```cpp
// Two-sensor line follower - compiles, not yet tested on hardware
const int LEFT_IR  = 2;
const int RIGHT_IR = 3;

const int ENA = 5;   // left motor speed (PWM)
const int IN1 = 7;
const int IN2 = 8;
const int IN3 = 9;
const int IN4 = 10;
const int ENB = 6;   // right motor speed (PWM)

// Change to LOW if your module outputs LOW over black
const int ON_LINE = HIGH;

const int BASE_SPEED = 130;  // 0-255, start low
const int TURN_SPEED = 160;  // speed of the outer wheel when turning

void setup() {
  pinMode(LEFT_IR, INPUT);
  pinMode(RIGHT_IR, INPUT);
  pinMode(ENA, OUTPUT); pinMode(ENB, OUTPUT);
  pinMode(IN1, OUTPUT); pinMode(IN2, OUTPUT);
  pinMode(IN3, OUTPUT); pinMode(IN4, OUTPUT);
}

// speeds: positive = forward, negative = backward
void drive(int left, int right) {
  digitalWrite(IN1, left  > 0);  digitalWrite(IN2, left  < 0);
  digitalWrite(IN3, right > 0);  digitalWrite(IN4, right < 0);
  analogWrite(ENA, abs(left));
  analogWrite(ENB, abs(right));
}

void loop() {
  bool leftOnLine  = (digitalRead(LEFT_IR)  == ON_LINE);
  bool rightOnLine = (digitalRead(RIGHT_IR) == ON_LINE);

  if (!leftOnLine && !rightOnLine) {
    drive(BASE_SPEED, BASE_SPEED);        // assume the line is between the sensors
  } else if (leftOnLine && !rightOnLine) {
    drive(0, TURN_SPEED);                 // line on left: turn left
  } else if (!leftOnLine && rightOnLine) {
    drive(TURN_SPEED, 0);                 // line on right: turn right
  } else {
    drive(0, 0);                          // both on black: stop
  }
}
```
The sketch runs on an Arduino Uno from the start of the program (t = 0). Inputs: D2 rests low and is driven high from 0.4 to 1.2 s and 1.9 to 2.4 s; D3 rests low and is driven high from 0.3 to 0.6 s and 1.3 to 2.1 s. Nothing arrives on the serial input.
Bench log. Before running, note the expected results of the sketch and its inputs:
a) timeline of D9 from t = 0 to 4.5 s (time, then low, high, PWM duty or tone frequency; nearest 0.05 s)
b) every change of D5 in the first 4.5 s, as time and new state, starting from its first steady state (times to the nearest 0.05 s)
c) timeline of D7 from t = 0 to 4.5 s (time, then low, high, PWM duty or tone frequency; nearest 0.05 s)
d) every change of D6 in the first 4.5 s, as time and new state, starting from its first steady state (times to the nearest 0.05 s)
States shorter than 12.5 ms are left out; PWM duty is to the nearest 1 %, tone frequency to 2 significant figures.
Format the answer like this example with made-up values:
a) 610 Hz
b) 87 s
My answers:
a) 0 s high; 0.3 s low; 0.6 s high; 1.3 s low; 2.1 s high
b) 0 s PWM 51 %; 0.3 s PWM 63 %; 0.4 s low; 1.2 s PWM 51 %; 1.3 s PWM 63 %; 1.9 s low; 2.4 s PWM 51 %
c) 0 s high; 0.4 s low; 1.2 s high; 1.9 s low; 2.4 s high
d) 0 s PWM 51 %; 0.3 s low; 0.6 s PWM 63 %; 1.2 s PWM 51 %; 1.3 s low; 2.1 s PWM 63 %; 2.4 s PWM 51 %
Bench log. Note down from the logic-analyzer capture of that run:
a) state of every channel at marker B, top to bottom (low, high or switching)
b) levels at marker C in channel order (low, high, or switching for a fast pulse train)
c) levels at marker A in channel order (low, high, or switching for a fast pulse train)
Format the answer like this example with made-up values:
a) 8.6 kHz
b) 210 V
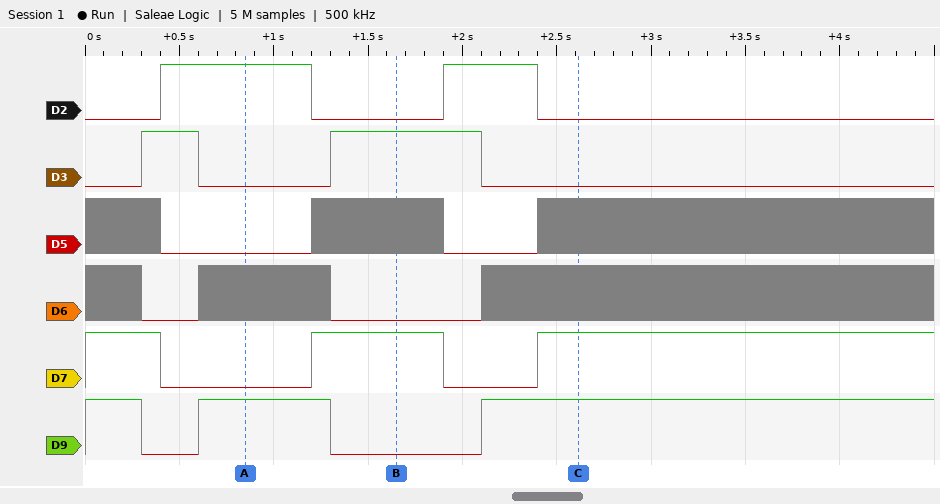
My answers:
a) D2 low, D3 high, D5 switching, D6 low, D7 high, D9 low
b) D2 low, D3 low, D5 switching, D6 switching, D7 high, D9 high
c) D2 high, D3 low, D5 low, D6 switching, D7 low, D9 high
